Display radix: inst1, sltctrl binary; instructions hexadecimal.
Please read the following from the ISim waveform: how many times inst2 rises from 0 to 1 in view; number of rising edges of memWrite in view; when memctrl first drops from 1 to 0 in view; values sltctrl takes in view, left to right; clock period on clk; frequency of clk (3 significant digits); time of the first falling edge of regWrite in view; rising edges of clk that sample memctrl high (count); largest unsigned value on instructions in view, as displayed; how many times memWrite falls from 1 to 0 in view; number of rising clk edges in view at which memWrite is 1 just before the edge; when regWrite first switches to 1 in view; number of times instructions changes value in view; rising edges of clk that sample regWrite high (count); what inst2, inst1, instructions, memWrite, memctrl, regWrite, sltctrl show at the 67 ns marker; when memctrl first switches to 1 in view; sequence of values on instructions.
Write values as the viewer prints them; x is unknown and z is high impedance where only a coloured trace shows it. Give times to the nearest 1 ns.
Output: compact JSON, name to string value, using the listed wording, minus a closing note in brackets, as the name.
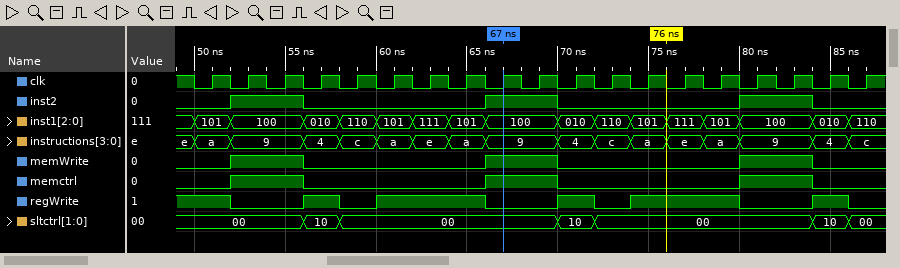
{"how many times inst2 rises from 0 to 1 in view": "3", "number of rising edges of memWrite in view": "3", "when memctrl first drops from 1 to 0 in view": "56 ns", "values sltctrl takes in view, left to right": "00, 10, 00, 10, 00, 10, 00", "clock period on clk": "2 ns", "frequency of clk": "500 MHz", "time of the first falling edge of regWrite in view": "52 ns", "rising edges of clk that sample memctrl high": "6", "largest unsigned value on instructions in view, as displayed": "e", "how many times memWrite falls from 1 to 0 in view": "3", "number of rising clk edges in view at which memWrite is 1 just before the edge": "6", "when regWrite first switches to 1 in view": "56 ns", "number of times instructions changes value in view": "16", "rising edges of clk that sample regWrite high": "10", "what inst2, inst1, instructions, memWrite, memctrl, regWrite, sltctrl show at the 67 ns marker": "inst2=1, inst1=100, instructions=9, memWrite=1, memctrl=1, regWrite=0, sltctrl=00", "when memctrl first switches to 1 in view": "52 ns", "sequence of values on instructions": "e, a, 9, 4, c, a, e, a, 9, 4, c, a, e, a, 9, 4, c"}
